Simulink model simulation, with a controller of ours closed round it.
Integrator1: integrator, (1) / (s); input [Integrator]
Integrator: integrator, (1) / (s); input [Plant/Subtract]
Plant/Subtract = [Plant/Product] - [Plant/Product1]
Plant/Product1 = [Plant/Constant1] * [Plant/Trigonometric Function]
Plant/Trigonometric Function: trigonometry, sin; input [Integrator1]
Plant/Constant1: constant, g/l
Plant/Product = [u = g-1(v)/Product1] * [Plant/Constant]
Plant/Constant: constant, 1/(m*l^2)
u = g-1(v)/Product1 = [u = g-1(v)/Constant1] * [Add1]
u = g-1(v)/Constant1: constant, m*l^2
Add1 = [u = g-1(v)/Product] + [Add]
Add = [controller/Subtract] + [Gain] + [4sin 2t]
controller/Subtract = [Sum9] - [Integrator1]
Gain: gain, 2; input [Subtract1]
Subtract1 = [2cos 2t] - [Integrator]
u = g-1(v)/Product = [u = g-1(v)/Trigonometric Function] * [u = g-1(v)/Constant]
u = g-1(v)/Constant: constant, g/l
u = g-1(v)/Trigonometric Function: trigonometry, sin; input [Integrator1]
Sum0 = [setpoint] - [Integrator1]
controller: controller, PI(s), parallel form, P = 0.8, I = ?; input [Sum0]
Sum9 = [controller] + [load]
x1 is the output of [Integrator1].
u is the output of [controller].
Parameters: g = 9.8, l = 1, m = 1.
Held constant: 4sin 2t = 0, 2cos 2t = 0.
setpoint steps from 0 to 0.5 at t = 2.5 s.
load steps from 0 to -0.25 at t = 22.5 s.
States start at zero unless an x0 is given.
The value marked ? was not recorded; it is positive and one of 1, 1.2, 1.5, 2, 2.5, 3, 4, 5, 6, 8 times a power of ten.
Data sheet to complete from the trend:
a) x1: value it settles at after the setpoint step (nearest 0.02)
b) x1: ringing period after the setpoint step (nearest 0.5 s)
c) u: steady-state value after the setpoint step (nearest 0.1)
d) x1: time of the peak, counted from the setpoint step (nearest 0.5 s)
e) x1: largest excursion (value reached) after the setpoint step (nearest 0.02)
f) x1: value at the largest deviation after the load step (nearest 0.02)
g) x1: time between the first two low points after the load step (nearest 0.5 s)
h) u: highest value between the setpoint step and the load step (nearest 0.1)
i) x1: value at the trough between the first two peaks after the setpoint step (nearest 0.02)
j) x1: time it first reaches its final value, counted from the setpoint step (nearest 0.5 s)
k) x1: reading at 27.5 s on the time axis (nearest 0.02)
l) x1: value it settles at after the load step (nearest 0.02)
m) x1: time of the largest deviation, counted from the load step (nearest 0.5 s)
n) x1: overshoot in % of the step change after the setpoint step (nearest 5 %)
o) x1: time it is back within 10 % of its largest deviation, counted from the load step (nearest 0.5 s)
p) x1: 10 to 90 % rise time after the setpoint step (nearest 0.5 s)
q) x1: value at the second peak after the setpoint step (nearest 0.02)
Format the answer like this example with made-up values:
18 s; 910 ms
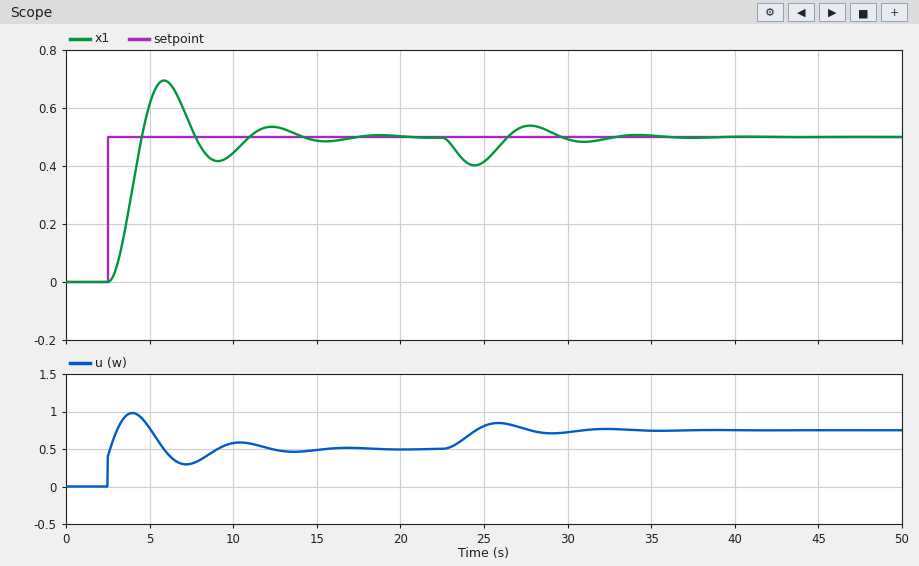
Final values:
0.50; 6.5 s; 0.5; 3.5 s; 0.70; 0.40; 6.5 s; 1.0; 0.42; 2.0 s; 0.54; 0.50; 2.0 s; 40 %; 9.5 s; 1.5 s; 0.54
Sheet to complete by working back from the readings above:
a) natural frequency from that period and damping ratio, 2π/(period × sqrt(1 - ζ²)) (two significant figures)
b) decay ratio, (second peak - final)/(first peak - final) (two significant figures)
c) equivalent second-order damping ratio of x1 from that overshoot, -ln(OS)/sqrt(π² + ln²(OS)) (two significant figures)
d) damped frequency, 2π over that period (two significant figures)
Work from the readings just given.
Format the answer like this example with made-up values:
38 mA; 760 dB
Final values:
1.0 rad/s; 0.20; 0.28; 0.97 rad/s
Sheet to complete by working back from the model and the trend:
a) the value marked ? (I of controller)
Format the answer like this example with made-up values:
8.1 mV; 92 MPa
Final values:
1.5
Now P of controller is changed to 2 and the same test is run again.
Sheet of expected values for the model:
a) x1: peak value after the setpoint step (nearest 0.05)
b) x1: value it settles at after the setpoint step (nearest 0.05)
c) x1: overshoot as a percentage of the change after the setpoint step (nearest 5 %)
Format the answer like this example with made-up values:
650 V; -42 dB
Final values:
0.60; 0.50; 20 %
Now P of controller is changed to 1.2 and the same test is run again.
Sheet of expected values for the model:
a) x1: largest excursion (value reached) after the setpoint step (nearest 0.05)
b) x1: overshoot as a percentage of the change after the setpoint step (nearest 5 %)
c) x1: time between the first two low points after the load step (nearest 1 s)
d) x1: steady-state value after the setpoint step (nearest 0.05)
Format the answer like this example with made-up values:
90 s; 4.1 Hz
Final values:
0.65; 30 %; 6 s; 0.50
